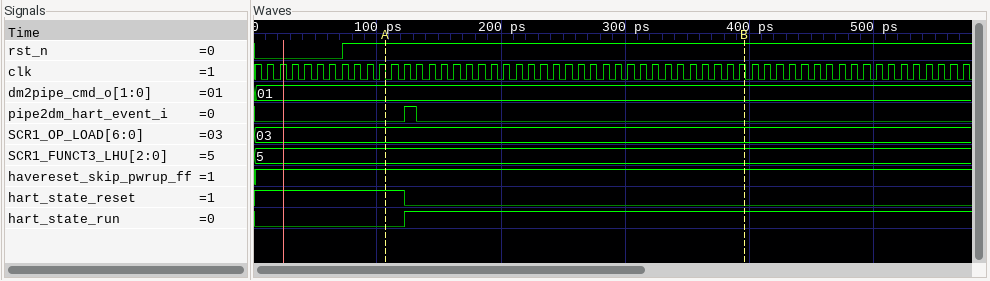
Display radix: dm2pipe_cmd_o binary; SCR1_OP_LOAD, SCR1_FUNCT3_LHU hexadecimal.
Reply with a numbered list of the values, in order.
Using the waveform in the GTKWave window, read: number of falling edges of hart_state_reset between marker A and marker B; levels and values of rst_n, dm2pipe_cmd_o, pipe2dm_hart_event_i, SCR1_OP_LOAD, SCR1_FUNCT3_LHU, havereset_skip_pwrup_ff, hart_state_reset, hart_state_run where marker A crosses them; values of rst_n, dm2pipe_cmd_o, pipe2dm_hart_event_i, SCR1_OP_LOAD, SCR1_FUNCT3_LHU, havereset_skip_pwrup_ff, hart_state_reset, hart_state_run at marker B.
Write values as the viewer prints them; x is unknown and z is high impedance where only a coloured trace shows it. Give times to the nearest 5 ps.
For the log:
1. 1
2. rst_n=1, dm2pipe_cmd_o=01, pipe2dm_hart_event_i=0, SCR1_OP_LOAD=03, SCR1_FUNCT3_LHU=5, havereset_skip_pwrup_ff=1, hart_state_reset=1, hart_state_run=0
3. rst_n=1, dm2pipe_cmd_o=01, pipe2dm_hart_event_i=0, SCR1_OP_LOAD=03, SCR1_FUNCT3_LHU=5, havereset_skip_pwrup_ff=1, hart_state_reset=0, hart_state_run=1
